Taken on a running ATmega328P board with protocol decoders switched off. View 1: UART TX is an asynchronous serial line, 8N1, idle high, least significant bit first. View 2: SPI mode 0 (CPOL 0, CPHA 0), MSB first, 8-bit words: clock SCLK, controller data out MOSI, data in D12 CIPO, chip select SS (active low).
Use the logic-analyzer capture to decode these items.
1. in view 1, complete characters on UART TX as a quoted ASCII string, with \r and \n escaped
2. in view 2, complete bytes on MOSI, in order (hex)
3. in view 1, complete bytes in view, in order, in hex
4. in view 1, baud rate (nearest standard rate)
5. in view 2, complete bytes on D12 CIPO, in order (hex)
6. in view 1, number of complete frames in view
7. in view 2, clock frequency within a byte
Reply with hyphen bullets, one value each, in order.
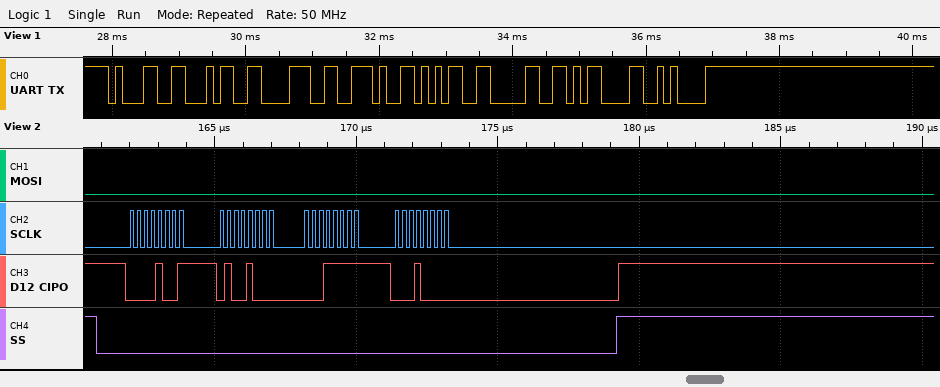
- "148.50\r\n"
- 0x00 0x00 0x00 0x00
- 31 34 38 2E 35 30 0D 0A
- 9600 baud
- 0x09 0x48 0x1F 0x10
- 8
- 4 MHz
